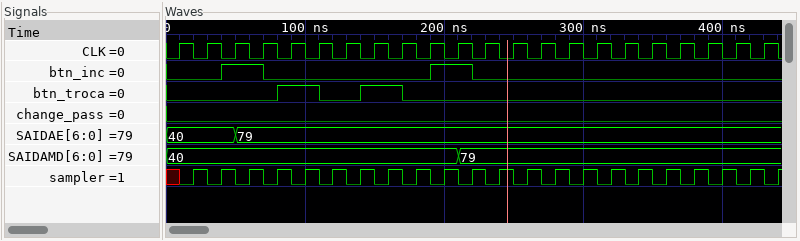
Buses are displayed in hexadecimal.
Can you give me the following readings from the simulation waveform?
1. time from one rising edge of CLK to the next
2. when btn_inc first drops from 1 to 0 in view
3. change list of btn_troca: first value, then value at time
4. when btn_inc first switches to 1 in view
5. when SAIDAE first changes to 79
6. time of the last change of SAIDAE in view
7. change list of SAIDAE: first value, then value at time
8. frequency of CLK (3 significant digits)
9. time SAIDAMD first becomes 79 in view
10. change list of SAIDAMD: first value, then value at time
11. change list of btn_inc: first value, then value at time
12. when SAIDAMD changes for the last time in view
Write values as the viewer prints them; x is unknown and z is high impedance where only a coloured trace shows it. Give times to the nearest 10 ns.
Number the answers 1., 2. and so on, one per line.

1. 20 ns
2. 70 ns
3. 0, 1 at 80 ns, 0 at 110 ns, 1 at 140 ns, 0 at 170 ns
4. 40 ns
5. 50 ns
6. 50 ns
7. 40, 79 at 50 ns
8. 50.0 MHz
9. 210 ns
10. 40, 79 at 210 ns
11. 0, 1 at 40 ns, 0 at 70 ns, 1 at 190 ns, 0 at 220 ns
12. 210 ns
